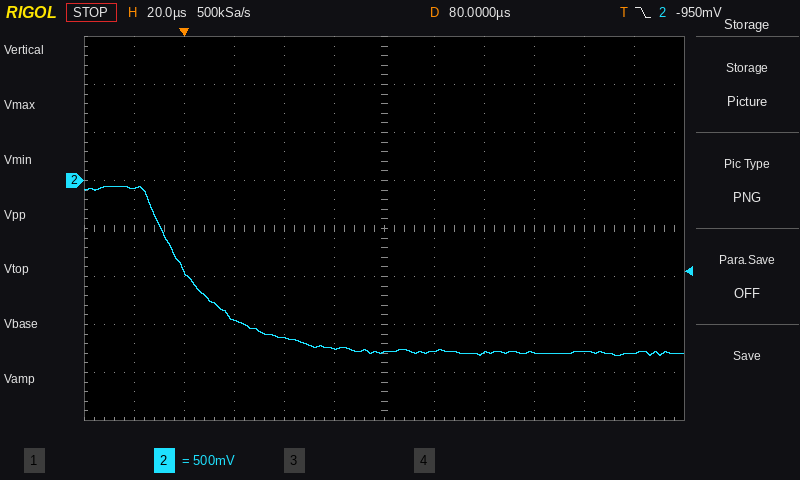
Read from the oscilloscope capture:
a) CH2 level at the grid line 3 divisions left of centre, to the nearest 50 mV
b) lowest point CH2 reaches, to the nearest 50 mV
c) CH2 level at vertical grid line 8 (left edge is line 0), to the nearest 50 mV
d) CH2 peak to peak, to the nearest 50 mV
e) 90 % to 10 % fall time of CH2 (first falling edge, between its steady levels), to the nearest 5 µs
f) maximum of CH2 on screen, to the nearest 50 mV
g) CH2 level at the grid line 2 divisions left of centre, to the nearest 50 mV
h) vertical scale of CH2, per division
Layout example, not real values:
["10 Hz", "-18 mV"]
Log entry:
["-1.45 V", "-1.80 V", "-1.80 V", "1.75 V", "50 µs", "-50 mV", "-1.65 V", "500 mV"]
